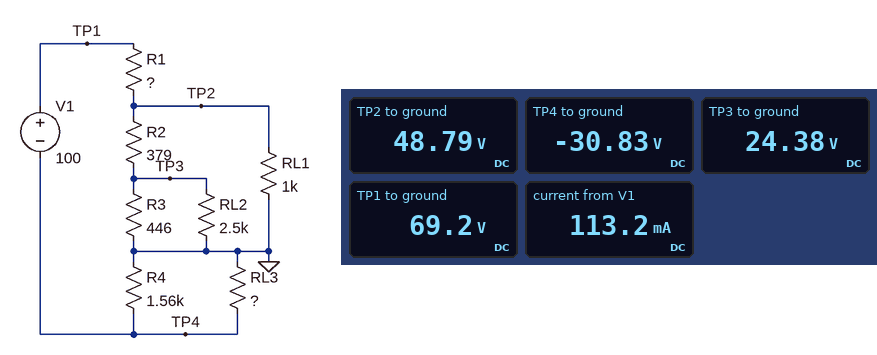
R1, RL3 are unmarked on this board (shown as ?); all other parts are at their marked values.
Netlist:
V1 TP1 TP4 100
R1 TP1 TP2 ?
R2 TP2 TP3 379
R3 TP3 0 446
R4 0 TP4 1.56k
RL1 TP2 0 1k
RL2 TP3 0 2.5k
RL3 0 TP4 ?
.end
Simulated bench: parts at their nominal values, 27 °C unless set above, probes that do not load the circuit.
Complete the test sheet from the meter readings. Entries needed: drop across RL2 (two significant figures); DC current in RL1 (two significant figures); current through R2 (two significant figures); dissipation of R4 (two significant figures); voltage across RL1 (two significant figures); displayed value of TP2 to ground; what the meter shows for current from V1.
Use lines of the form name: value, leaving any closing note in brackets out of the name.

drop across RL2: 24 V
DC current in RL1: 49 mA
current through R2: 64 mA
dissipation of R4: 610 mW
voltage across RL1: 49 V
displayed value of TP2 to ground: 48.79 V
what the meter shows for current from V1: 113.2 mA
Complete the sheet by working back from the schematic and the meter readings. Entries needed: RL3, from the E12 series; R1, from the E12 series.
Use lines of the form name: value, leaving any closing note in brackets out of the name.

RL3, from the E12 series: 330 Ω
R1, from the E12 series: 180 Ω
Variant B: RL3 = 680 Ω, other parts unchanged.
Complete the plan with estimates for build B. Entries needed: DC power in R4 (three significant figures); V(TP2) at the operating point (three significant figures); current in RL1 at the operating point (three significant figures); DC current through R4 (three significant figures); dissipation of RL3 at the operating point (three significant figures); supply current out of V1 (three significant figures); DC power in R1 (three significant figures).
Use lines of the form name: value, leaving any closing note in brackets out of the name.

DC power in R4: 1.22 W
V(TP2) at the operating point: 39.7 V
current in RL1 at the operating point: 39.7 mA
DC current through R4: 28.0 mA
dissipation of RL3 at the operating point: 2.80 W
supply current out of V1: 92.2 mA
DC power in R1: 1.53 W
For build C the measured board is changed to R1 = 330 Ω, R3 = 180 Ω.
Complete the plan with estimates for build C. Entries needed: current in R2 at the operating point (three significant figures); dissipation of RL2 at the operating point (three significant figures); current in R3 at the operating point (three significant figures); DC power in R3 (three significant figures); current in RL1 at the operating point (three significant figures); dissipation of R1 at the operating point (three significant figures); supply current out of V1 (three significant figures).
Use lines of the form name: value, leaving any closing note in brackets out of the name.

current in R2 at the operating point: 67.6 mA
dissipation of RL2 at the operating point: 51.6 mW
current in R3 at the operating point: 63.1 mA
DC power in R3: 716 mW
current in RL1 at the operating point: 37.0 mA
dissipation of R1 at the operating point: 3.61 W
supply current out of V1: 105 mA
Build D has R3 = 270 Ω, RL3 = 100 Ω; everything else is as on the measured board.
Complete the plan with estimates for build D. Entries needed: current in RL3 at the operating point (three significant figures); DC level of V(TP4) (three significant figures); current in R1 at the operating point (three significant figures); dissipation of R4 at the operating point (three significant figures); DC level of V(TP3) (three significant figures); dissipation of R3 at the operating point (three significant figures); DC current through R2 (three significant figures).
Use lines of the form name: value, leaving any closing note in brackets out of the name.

current in RL3 at the operating point: 143 mA
DC level of V(TP4): -14.3 V
current in R1 at the operating point: 152 mA
dissipation of R4 at the operating point: 131 mW
DC level of V(TP3): 22.8 V
dissipation of R3 at the operating point: 1.93 W
DC current through R2: 93.7 mA
